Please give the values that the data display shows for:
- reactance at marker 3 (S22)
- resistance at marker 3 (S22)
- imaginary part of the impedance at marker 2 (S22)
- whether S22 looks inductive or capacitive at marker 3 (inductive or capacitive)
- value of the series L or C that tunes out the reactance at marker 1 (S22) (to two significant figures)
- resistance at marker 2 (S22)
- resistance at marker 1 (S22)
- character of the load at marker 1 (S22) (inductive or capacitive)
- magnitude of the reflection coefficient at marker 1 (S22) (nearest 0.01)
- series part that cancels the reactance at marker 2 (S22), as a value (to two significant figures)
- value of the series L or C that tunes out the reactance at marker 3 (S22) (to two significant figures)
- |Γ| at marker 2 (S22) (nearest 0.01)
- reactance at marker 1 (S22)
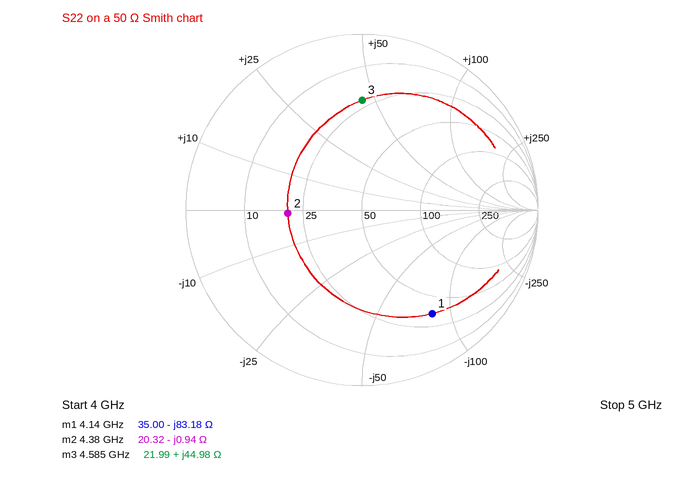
+44.98 Ω
21.99 Ω
-0.94 Ω
inductive
3.2 nH
20.32 Ω
35.00 Ω
capacitive
0.71
34 pH
770 fF
0.42
-83.18 Ω
